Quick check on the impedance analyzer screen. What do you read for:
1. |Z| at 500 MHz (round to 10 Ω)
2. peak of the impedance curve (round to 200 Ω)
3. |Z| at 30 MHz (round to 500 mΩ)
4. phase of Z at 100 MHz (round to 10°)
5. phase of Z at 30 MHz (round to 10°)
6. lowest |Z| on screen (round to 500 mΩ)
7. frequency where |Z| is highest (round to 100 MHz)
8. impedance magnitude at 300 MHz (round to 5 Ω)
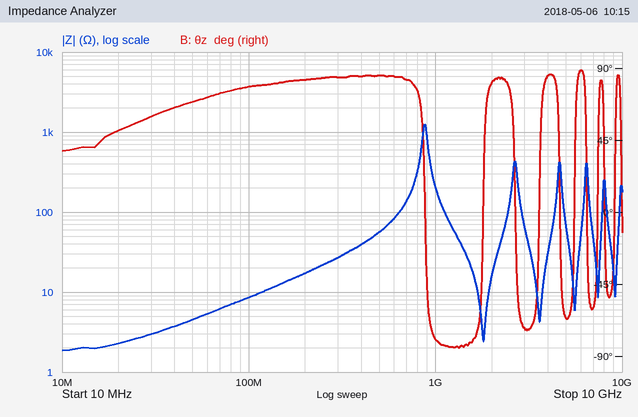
60 Ω
1.2 kΩ
3.0 Ω
80°
60°
2.0 Ω
900 MHz
25 Ω
